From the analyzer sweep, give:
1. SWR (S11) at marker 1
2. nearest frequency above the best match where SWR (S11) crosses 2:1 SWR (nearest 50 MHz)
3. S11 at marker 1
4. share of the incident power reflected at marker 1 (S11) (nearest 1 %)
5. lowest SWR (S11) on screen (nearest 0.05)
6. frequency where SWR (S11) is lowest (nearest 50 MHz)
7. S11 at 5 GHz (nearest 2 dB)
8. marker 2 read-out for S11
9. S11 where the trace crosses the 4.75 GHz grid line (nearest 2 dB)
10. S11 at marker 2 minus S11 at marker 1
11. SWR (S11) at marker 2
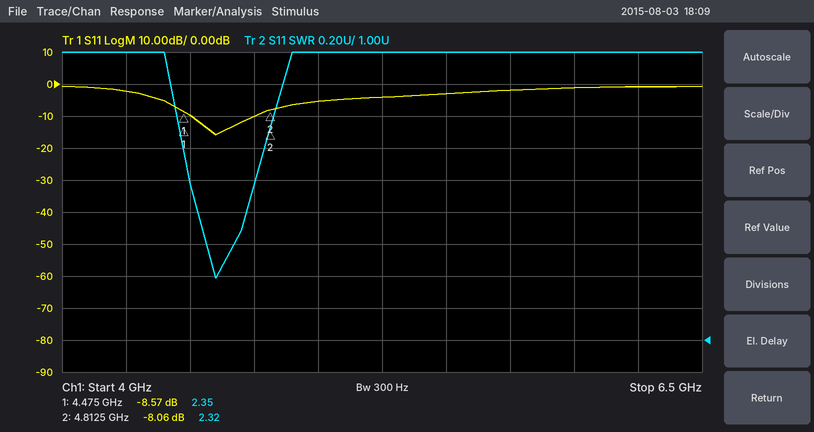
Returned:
2.35
4.75 GHz
-8.57 dB
14 %
1.40
4.60 GHz
-6 dB
-8.06 dB
-10 dB
0.51 dB
2.32
